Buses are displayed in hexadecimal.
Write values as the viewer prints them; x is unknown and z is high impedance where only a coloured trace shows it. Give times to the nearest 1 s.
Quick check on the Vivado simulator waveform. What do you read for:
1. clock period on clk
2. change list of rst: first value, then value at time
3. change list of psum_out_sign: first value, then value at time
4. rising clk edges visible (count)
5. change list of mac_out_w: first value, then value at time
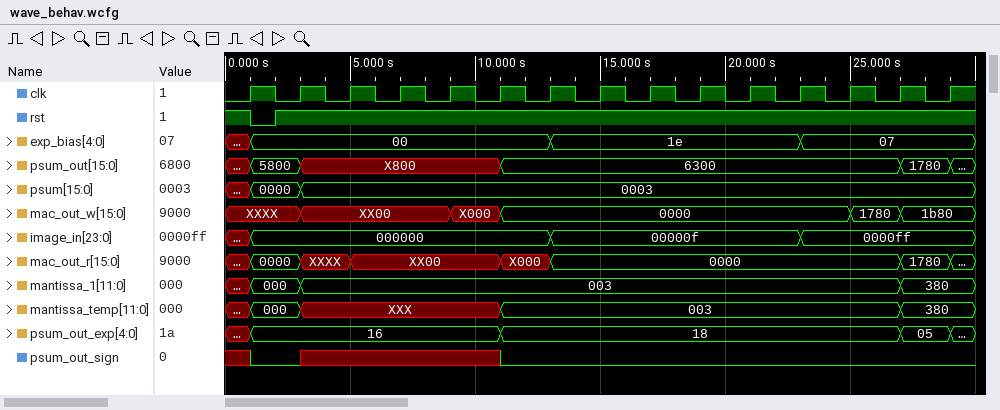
2 s
1, 0 at 1 s, 1 at 2 s
x, 0 at 1 s, x at 3 s, 0 at 11 s
15
XXXX, XX00 at 3 s, X000 at 9 s, 0000 at 11 s, 1780 at 25 s, 1b80 at 27 s
